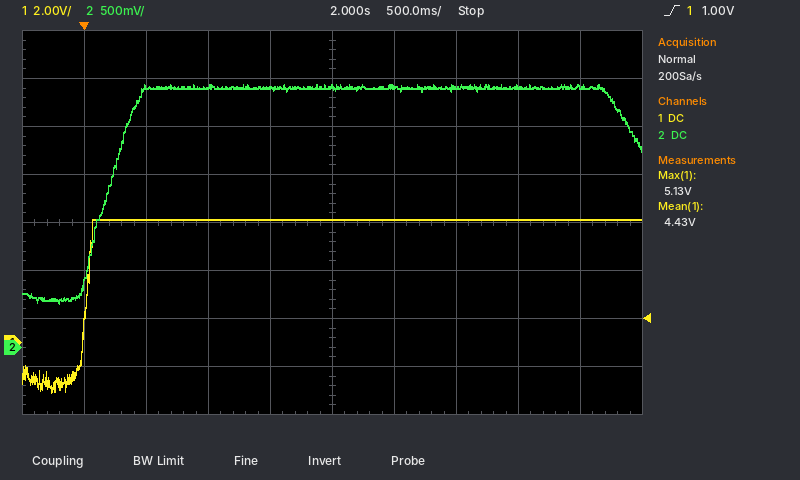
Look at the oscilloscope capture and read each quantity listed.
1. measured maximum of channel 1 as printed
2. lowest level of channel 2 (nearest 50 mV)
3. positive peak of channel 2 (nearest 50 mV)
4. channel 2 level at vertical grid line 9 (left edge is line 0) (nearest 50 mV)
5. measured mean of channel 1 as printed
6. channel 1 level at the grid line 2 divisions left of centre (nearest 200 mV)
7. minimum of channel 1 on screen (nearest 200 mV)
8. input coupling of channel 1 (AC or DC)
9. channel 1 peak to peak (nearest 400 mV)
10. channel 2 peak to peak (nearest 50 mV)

5.13 V
450 mV
2.75 V
2.70 V
4.43 V
5.2 V
-2.0 V
DC
7.2 V
2.30 V
